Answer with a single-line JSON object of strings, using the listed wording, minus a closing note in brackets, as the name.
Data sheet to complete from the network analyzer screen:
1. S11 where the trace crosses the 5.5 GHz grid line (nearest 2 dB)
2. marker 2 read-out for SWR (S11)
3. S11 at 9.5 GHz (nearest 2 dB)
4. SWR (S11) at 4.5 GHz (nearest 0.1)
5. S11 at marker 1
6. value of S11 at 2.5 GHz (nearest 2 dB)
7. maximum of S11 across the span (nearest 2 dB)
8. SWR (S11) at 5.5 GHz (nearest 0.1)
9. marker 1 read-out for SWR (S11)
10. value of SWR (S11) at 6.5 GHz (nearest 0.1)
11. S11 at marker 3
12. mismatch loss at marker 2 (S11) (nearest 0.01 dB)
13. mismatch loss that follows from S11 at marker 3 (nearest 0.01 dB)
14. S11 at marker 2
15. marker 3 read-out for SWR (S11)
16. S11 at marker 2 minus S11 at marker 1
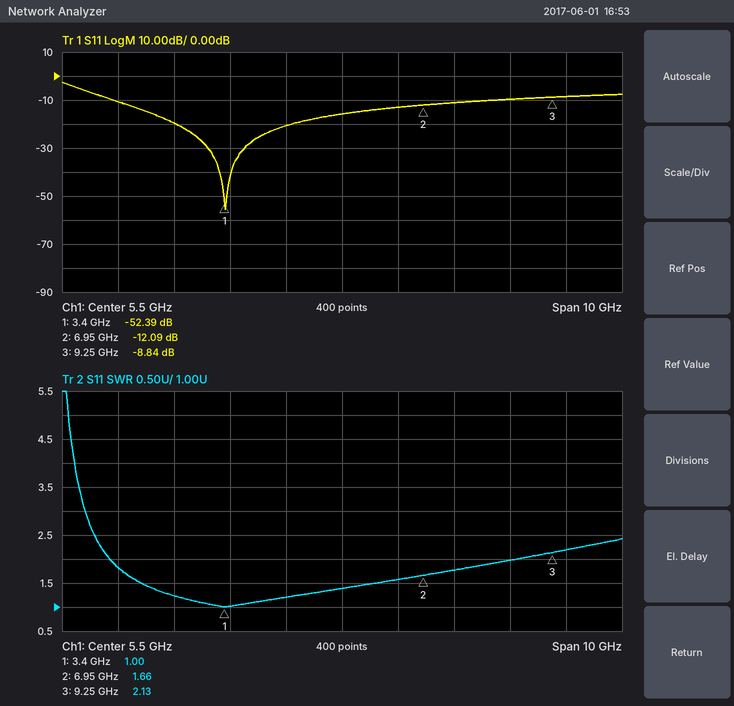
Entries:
{"S11 where the trace crosses the 5.5 GHz grid line": "-16 dB", "marker 2 read-out for SWR": "1.66", "S11 at 9.5 GHz": "-8 dB", "SWR (S11) at 4.5 GHz": "1.2", "S11 at marker 1": "-52.39 dB", "value of S11 at 2.5 GHz": "-20 dB", "maximum of S11 across the span": "-2 dB", "SWR (S11) at 5.5 GHz": "1.4", "marker 1 read-out for SWR": "1.00", "value of SWR (S11) at 6.5 GHz": "1.6", "S11 at marker 3": "-8.84 dB", "mismatch loss at marker 2 (S11)": "0.28 dB", "mismatch loss that follows from S11 at marker 3": "0.61 dB", "S11 at marker 2": "-12.09 dB", "marker 3 read-out for SWR": "2.13", "S11 at marker 2 minus S11 at marker 1": "40.30 dB"}
